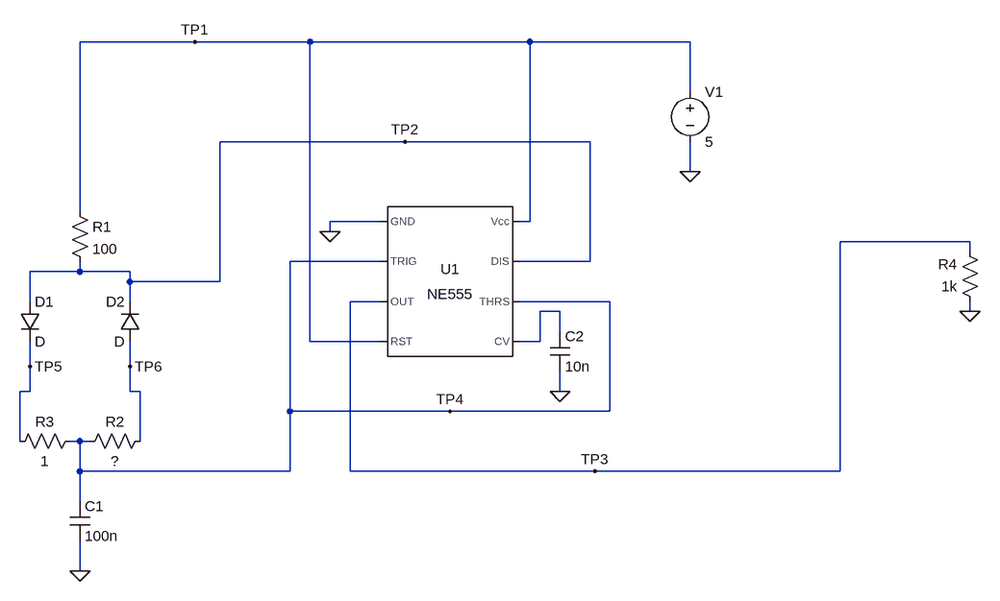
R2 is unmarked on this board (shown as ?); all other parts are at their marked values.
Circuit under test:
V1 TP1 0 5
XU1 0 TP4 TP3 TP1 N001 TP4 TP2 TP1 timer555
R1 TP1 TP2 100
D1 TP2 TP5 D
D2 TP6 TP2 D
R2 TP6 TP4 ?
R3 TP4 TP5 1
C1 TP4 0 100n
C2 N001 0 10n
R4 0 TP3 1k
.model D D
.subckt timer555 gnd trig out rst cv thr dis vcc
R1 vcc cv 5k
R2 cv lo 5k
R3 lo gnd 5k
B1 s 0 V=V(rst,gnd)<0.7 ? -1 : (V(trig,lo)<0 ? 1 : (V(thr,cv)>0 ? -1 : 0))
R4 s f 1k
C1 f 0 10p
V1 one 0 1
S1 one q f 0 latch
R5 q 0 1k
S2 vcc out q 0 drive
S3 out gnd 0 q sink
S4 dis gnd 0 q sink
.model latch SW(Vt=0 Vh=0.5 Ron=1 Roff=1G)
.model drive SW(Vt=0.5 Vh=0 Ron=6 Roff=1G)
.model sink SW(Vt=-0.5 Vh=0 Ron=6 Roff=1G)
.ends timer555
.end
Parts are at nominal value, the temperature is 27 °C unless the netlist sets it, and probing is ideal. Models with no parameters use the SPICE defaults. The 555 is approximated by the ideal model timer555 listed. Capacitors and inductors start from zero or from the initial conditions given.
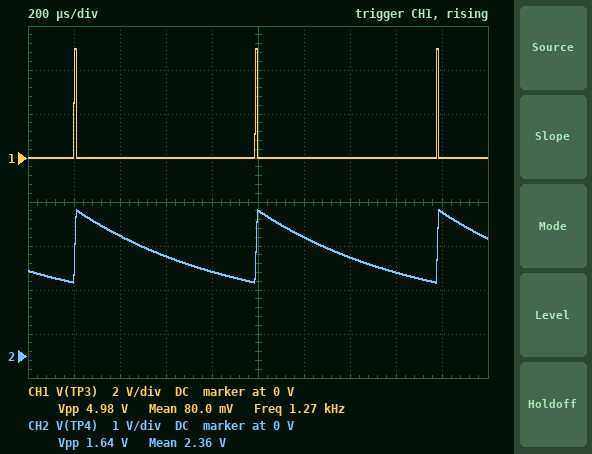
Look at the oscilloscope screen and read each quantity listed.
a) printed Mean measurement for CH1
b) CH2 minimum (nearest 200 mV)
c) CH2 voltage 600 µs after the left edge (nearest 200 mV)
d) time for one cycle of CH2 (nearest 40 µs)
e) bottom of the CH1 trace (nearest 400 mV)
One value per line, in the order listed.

80.0 mV
1.6 V
2.2 V
800 µs
0 V
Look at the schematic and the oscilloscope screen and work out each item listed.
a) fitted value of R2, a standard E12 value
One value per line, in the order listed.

6.8 kΩ
